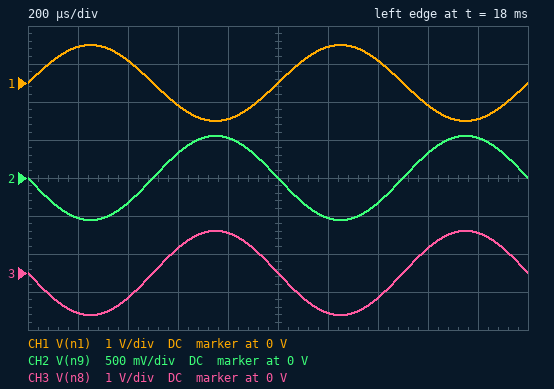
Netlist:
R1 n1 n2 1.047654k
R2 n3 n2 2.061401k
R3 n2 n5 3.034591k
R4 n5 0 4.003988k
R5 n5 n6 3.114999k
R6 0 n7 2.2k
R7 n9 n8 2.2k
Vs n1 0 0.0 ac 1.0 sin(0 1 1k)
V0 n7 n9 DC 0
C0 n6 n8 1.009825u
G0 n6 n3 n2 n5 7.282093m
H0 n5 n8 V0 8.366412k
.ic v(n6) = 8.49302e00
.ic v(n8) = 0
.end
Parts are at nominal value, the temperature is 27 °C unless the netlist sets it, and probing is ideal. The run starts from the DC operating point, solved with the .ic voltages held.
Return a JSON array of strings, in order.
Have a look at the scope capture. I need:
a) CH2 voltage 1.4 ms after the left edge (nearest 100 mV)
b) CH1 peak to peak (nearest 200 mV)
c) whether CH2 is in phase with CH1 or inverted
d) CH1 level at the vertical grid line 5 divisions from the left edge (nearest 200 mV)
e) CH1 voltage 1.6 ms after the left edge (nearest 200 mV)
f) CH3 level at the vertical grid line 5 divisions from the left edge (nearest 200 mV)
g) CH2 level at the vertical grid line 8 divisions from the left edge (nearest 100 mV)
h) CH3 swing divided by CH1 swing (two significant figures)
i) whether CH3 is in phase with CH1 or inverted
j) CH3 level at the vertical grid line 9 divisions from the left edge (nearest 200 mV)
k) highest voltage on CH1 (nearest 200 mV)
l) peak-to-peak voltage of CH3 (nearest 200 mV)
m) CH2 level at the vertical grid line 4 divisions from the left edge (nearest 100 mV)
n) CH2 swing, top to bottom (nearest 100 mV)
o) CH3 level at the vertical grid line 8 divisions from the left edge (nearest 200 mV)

["-300 mV", "2.0 V", "inverted", "0 V", "-600 mV", "0 V", "300 mV", "1.1", "inverted", "1.0 V", "1.0 V", "2.2 V", "500 mV", "1.1 V", "600 mV"]
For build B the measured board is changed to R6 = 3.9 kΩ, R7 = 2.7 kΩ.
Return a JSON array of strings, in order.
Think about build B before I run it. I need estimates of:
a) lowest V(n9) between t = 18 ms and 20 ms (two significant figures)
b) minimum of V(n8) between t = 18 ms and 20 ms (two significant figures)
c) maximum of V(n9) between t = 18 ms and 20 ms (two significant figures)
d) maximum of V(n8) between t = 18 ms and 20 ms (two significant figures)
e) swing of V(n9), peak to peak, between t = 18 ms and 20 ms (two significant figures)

["-3.1 V", "-5.2 V", "3.1 V", "5.2 V", "6.2 V"]
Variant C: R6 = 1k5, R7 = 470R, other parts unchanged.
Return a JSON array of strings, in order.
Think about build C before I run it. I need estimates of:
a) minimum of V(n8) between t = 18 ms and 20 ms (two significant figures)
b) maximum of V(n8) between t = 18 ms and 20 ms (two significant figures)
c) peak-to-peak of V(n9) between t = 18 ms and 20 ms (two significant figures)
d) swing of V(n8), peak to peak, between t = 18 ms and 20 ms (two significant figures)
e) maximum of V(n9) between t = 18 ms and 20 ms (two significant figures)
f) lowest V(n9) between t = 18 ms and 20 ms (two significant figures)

["-280 mV", "280 mV", "430 mV", "570 mV", "220 mV", "-220 mV"]
